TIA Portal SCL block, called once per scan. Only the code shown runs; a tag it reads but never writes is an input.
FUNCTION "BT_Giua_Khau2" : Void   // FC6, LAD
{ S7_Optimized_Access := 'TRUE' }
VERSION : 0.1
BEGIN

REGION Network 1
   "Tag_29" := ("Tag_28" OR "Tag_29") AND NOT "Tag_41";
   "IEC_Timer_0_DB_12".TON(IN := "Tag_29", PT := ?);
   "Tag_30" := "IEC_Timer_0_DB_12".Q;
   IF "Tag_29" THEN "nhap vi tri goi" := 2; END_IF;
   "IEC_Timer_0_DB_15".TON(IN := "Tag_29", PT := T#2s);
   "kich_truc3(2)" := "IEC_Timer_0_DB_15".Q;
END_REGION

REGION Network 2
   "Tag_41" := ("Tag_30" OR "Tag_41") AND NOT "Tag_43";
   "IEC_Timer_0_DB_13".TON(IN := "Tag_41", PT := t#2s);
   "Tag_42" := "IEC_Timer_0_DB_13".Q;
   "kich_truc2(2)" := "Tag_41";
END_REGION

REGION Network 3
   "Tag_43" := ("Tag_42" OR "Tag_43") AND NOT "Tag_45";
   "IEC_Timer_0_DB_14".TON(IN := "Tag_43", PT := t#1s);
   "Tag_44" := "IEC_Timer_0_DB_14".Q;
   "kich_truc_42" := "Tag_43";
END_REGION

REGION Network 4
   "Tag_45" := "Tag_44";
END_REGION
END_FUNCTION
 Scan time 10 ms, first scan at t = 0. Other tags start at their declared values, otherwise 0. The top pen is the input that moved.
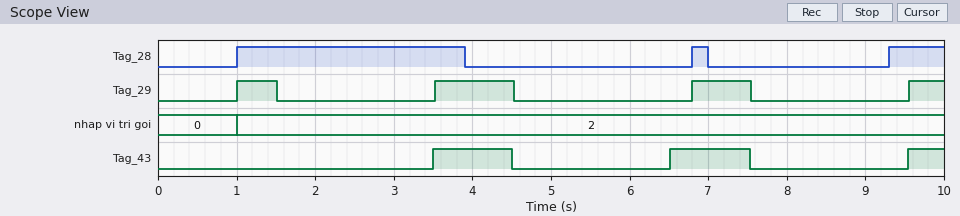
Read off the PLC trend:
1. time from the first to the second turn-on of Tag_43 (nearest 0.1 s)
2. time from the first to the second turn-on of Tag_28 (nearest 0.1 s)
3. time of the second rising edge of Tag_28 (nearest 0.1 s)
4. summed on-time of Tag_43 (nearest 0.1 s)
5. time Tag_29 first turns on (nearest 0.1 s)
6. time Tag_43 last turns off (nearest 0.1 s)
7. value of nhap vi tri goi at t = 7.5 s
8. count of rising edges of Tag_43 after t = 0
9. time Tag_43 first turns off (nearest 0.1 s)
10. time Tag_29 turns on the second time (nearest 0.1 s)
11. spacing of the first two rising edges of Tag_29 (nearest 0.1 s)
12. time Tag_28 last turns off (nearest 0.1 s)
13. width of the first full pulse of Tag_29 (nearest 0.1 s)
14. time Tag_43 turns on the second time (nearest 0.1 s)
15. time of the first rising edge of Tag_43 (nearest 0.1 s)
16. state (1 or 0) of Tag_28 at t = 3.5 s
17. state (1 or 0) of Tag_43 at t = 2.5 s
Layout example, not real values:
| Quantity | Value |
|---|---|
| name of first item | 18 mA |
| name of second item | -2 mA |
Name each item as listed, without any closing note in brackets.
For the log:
| Quantity | Value |
|---|---|
| time from the first to the second turn-on of Tag_43 | 3.0 s |
| time from the first to the second turn-on of Tag_28 | 5.8 s |
| time of the second rising edge of Tag_28 | 6.8 s |
| summed on-time of Tag_43 | 2.5 s |
| time Tag_29 first turns on | 1.0 s |
| time Tag_43 last turns off | 7.5 s |
| value of nhap vi tri goi at t = 7.5 s | 2 |
| count of rising edges of Tag_43 after t = 0 | 3 |
| time Tag_43 first turns off | 4.5 s |
| time Tag_29 turns on the second time | 3.5 s |
| spacing of the first two rising edges of Tag_29 | 2.5 s |
| time Tag_28 last turns off | 7.0 s |
| width of the first full pulse of Tag_29 | 0.5 s |
| time Tag_43 turns on the second time | 6.5 s |
| time of the first rising edge of Tag_43 | 3.5 s |
| state (1 or 0) of Tag_28 at t = 3.5 s | 1 |
| state (1 or 0) of Tag_43 at t = 2.5 s | 0 |
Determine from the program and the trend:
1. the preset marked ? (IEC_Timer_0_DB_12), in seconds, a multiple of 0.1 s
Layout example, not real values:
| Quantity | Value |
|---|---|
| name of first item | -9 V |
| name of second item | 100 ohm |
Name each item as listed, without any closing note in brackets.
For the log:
| Quantity | Value |
|---|---|
| the preset marked ? (IEC_Timer_0_DB_12), in seconds, a multiple of 0.1 s | 0.5 s |
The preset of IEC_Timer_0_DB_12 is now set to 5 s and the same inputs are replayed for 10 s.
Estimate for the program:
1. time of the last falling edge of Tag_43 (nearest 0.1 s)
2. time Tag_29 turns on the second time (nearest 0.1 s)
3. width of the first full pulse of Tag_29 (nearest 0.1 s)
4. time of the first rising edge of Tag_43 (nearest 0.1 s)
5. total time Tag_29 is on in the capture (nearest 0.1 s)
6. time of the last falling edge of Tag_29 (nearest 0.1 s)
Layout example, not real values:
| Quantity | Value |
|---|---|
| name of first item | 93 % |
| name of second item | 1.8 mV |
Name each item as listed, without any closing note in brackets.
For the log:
| Quantity | Value |
|---|---|
| time of the last falling edge of Tag_43 | 9.0 s |
| time Tag_29 turns on the second time | 9.3 s |
| width of the first full pulse of Tag_29 | 5.0 s |
| time of the first rising edge of Tag_43 | 8.0 s |
| total time Tag_29 is on in the capture | 5.7 s |
| time of the last falling edge of Tag_29 | 6.0 s |
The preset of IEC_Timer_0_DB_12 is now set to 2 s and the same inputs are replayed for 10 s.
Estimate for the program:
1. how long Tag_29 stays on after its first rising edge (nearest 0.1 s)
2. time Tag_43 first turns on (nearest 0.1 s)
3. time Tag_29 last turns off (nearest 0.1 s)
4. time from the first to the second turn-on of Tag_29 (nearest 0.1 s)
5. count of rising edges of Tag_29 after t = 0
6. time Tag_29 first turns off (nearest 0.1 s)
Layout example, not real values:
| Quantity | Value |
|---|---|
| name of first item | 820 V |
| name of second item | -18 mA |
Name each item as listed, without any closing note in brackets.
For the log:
| Quantity | Value |
|---|---|
| how long Tag_29 stays on after its first rising edge | 2.0 s |
| time Tag_43 first turns on | 5.0 s |
| time Tag_29 last turns off | 8.8 s |
| time from the first to the second turn-on of Tag_29 | 5.8 s |
| count of rising edges of Tag_29 after t = 0 | 2 |
| time Tag_29 first turns off | 3.0 s |
